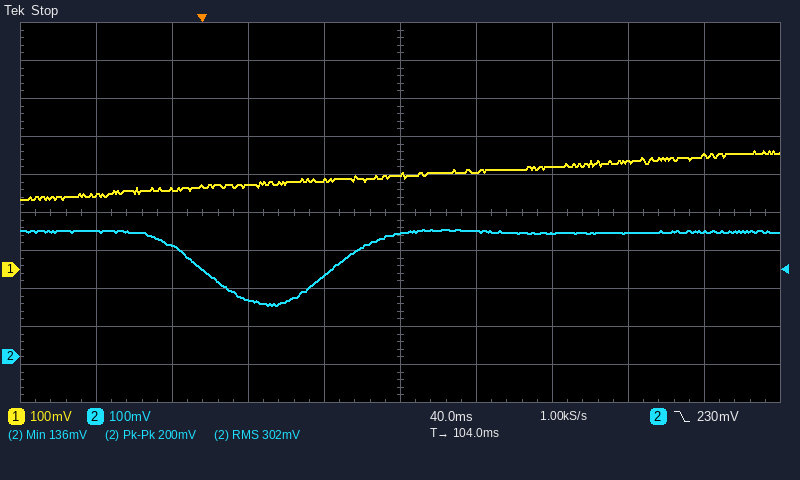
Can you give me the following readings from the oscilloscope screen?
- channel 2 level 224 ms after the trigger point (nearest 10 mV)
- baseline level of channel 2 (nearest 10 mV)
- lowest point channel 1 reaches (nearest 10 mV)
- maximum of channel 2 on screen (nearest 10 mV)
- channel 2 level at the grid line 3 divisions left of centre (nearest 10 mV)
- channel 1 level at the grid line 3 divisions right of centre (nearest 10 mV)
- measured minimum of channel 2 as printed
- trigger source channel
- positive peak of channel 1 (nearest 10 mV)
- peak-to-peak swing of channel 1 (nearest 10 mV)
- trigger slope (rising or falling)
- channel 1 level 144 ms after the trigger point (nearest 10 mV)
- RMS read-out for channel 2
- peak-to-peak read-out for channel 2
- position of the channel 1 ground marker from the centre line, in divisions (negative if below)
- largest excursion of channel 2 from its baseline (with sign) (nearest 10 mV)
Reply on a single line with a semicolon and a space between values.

330 mV; 330 mV; 180 mV; 340 mV; 290 mV; 280 mV; 136 mV; channel 2; 310 mV; 130 mV; falling; 260 mV; 302 mV; 200 mV; -1.5 div; -190 mV
